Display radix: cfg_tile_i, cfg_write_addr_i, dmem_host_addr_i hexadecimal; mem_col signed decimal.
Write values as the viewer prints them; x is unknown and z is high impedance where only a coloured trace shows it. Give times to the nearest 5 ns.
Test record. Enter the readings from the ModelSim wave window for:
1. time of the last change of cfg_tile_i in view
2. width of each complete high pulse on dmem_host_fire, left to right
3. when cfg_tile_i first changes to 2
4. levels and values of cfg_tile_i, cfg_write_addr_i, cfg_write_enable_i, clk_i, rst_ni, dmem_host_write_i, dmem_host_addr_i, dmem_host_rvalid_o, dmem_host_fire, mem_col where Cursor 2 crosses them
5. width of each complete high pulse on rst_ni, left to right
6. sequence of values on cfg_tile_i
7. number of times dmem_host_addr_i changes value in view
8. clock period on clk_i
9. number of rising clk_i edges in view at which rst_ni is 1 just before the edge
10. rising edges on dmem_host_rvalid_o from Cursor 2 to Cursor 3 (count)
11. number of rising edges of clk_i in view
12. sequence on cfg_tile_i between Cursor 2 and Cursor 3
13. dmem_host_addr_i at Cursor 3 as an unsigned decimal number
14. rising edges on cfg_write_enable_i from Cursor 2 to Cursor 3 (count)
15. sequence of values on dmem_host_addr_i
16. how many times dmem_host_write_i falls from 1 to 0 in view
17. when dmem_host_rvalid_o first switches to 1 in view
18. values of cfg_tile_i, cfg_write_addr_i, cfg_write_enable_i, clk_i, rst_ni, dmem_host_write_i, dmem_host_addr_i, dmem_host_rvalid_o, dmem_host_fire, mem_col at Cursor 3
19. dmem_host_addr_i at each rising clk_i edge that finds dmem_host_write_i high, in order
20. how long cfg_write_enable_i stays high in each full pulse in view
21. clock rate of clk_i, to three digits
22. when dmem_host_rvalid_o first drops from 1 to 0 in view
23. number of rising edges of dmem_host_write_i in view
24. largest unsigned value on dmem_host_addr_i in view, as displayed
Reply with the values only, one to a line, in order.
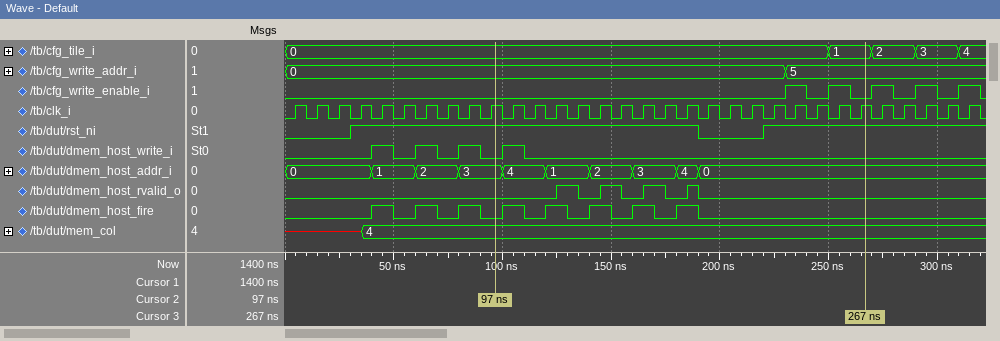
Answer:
310 ns
10 ns, 10 ns, 10 ns, 10 ns, 10 ns, 10 ns, 10 ns, 10 ns
270 ns
cfg_tile_i=0, cfg_write_addr_i=0, cfg_write_enable_i=0, clk_i=1, rst_ni=1, dmem_host_write_i=0, dmem_host_addr_i=3, dmem_host_rvalid_o=0, dmem_host_fire=0, mem_col=4
160 ns
0, 1, 2, 3, 4
9
10 ns
26
4
32
0, 1
0
2
0, 1, 2, 3, 4, 1, 2, 3, 4, 0
4
125 ns
cfg_tile_i=1, cfg_write_addr_i=5, cfg_write_enable_i=0, clk_i=1, rst_ni=1, dmem_host_write_i=0, dmem_host_addr_i=0, dmem_host_rvalid_o=0, dmem_host_fire=0, mem_col=4
1, 2, 3, 4
10 ns, 10 ns, 10 ns, 10 ns, 10 ns
100 MHz
135 ns
4
4
